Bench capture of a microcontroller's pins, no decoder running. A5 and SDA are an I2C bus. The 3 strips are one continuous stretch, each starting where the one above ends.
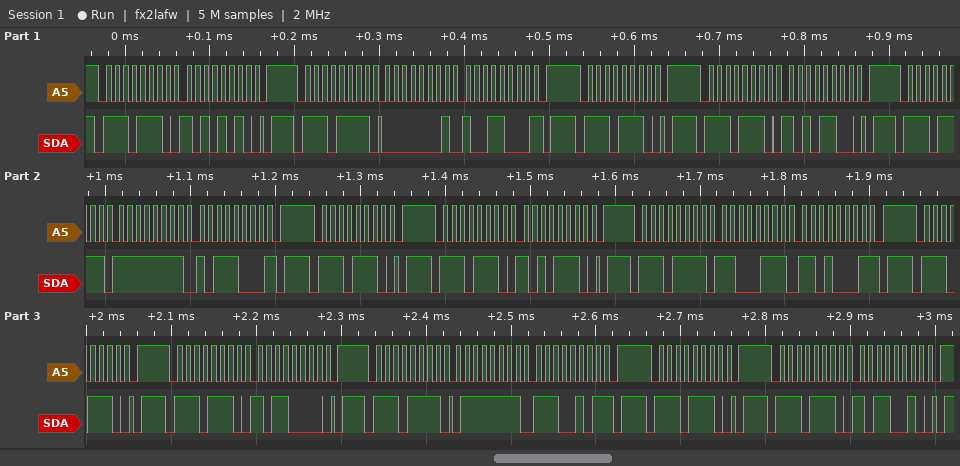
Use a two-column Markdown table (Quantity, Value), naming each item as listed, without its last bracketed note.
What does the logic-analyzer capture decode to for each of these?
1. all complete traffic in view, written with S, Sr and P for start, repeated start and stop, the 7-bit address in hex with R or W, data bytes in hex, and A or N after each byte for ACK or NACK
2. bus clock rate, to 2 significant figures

| Quantity | Value |
|---|---|
| all complete traffic in view, written with S, Sr and P for start, repeated start and stop, the 7-bit address in hex with R or W, data bytes in hex, and A or N after each byte for ACK or NACK | S 77W A AA A P S 77R A 01 A 98 N P S 77W A P S 77W A AC A P S 77R A FF A B8 N P S 77W A P S 77W A AE A P S 77R A C7 A D1 N P S 77W A P S 77W A B0 A P S 77R A 7F A E5 N P S 77W A P S 77W A B2 A P |
| bus clock rate, to 2 significant figures | 100 kHz |
